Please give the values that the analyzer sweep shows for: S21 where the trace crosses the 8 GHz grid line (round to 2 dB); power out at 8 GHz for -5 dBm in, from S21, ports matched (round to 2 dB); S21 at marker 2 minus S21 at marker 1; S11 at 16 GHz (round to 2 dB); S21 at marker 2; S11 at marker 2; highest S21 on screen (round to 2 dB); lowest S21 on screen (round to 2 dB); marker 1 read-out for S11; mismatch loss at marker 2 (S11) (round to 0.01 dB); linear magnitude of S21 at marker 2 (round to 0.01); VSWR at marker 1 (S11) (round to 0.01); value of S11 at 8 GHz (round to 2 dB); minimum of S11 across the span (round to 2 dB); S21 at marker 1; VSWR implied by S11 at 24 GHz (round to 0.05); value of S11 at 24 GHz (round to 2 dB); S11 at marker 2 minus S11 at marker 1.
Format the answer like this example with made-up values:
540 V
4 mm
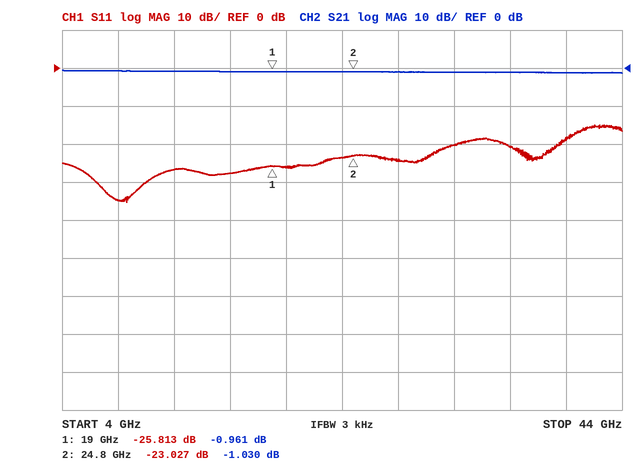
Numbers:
0 dB
-6 dBm
-0.069 dB
-28 dB
-1.030 dB
-23.027 dB
0 dB
-2 dB
-25.813 dB
0.02 dB
0.89
1.11
-34 dB
-36 dB
-0.961 dB
1.15
-24 dB
2.786 dB
